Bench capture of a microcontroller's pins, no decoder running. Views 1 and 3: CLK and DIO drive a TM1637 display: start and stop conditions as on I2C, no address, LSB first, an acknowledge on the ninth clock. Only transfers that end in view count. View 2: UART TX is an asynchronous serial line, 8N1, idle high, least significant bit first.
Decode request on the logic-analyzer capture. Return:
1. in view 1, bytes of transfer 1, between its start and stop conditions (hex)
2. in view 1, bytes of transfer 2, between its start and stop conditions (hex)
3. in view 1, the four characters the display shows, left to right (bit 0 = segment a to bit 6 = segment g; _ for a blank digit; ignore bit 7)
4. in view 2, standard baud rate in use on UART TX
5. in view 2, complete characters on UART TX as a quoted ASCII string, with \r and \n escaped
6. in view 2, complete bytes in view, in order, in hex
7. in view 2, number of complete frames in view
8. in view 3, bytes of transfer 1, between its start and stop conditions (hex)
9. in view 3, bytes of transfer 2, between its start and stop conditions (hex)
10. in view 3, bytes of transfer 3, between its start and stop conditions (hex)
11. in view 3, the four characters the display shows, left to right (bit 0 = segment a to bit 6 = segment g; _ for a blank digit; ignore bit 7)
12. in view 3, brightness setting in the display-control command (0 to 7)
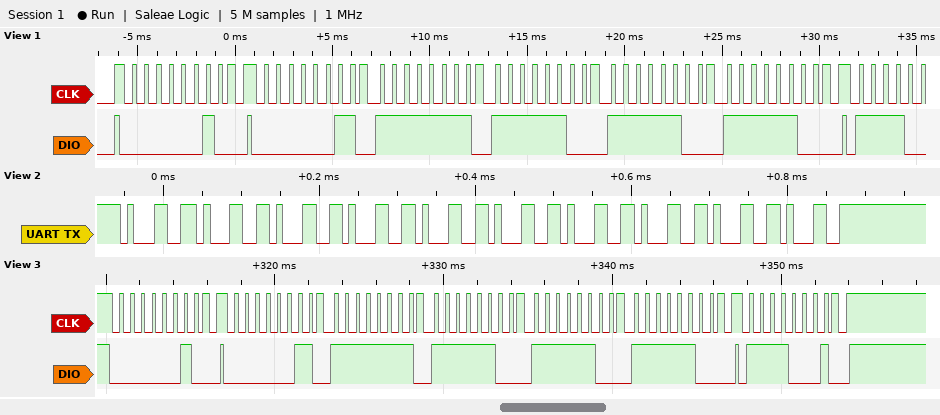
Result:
40
C0 FF 3F 3F 3F
8000
115200 baud
"1111111111"
31 31 31 31 31 31 31 31 31 31
10
40
C0 FF 3F 3F 3F
8F
8000
7
